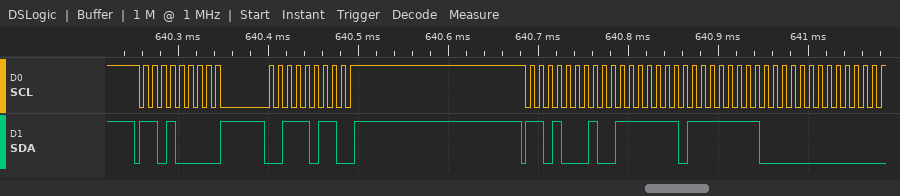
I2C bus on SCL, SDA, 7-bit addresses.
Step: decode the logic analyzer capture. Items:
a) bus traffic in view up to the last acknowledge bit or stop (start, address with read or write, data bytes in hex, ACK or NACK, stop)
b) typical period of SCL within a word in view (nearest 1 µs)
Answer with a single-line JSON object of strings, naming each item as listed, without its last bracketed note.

{"bus traffic in view up to the last acknowledge bit or stop": "start, address 68 write ACK, 3B ACK, stop, start, address 68 read ACK, 7F ACK, FF ACK, 00 ACK", "typical period of SCL within a word in view": "10 µs"}
